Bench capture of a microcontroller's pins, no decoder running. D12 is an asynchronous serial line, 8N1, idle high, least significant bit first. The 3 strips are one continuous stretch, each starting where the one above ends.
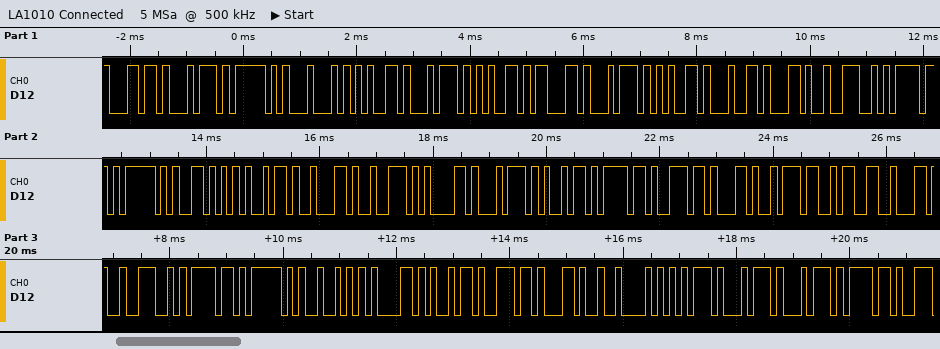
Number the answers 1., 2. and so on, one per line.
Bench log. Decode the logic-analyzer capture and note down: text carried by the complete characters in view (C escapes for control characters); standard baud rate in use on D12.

1. "lt_Detected,No_Vibration,73,No_Rain,Butto"
2. 9600 baud
